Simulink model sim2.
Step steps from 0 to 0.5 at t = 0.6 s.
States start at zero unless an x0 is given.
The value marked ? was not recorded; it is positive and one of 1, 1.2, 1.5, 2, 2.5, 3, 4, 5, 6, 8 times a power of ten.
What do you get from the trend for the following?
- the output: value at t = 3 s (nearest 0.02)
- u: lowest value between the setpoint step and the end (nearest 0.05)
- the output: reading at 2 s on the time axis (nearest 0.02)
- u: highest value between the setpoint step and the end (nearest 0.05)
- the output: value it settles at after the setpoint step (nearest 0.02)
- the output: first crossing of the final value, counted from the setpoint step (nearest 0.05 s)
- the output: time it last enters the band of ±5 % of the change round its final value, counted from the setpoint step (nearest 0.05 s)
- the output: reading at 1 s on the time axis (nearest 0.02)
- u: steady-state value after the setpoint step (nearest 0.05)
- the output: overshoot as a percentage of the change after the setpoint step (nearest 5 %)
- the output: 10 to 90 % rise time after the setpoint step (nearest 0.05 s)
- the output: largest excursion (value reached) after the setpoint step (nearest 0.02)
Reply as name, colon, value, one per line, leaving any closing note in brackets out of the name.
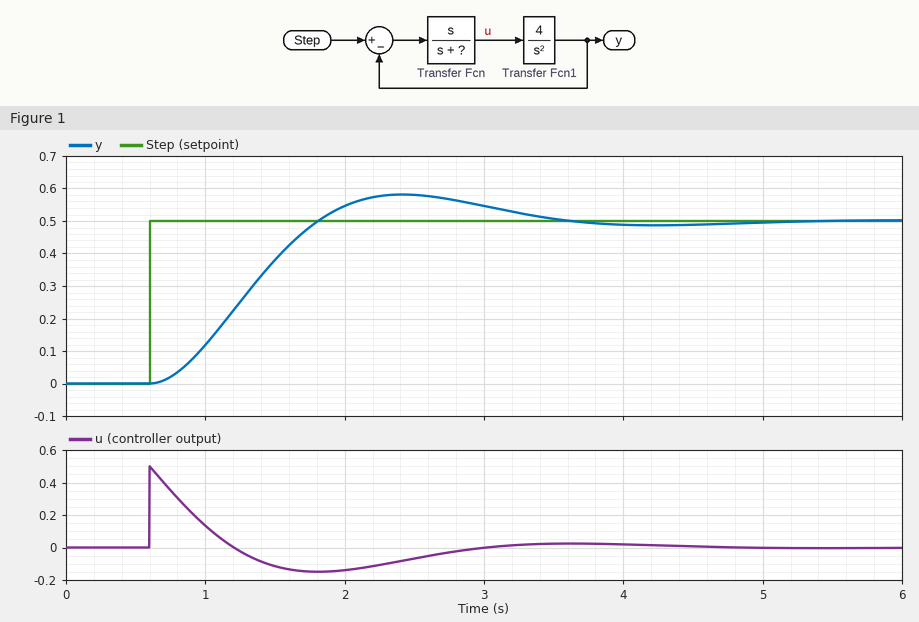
the output: value at t = 3 s: 0.54
u: lowest value between the setpoint step and the end: -0.15
the output: reading at 2 s on the time axis: 0.54
u: highest value between the setpoint step and the end: 0.50
the output: value it settles at after the setpoint step: 0.50
the output: first crossing of the final value, counted from the setpoint step: 1.20 s
the output: time it last enters the band of ±5 % of the change round its final value, counted from the setpoint step: 2.65 s
the output: reading at 1 s on the time axis: 0.12
u: steady-state value after the setpoint step: 0.00
the output: overshoot as a percentage of the change after the setpoint step: 15 %
the output: 10 to 90 % rise time after the setpoint step: 0.80 s
the output: largest excursion (value reached) after the setpoint step: 0.58
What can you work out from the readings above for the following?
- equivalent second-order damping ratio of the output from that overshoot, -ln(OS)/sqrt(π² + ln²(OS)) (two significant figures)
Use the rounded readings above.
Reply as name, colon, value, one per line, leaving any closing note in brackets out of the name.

equivalent second-order damping ratio of the output from that overshoot, -ln(OS)/sqrt(π² + ln²(OS)): 0.52
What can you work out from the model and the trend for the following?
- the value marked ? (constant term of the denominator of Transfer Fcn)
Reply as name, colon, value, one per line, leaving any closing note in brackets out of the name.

the value marked ?: 2
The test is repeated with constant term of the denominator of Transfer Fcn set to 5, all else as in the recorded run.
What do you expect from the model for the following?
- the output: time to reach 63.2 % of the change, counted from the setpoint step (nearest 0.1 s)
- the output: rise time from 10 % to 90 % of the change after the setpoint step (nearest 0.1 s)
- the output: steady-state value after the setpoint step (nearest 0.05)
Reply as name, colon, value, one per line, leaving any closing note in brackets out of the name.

the output: time to reach 63.2 % of the change, counted from the setpoint step: 1.3 s
the output: rise time from 10 % to 90 % of the change after the setpoint step: 2.3 s
the output: steady-state value after the setpoint step: 0.50
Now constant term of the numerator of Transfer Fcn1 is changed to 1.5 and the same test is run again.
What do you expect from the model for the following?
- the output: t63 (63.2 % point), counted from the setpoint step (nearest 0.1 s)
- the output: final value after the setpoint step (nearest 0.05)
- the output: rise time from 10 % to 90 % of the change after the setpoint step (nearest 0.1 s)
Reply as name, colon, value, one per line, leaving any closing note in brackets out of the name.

the output: t63 (63.2 % point), counted from the setpoint step: 1.5 s
the output: final value after the setpoint step: 0.50
the output: rise time from 10 % to 90 % of the change after the setpoint step: 2.1 s
